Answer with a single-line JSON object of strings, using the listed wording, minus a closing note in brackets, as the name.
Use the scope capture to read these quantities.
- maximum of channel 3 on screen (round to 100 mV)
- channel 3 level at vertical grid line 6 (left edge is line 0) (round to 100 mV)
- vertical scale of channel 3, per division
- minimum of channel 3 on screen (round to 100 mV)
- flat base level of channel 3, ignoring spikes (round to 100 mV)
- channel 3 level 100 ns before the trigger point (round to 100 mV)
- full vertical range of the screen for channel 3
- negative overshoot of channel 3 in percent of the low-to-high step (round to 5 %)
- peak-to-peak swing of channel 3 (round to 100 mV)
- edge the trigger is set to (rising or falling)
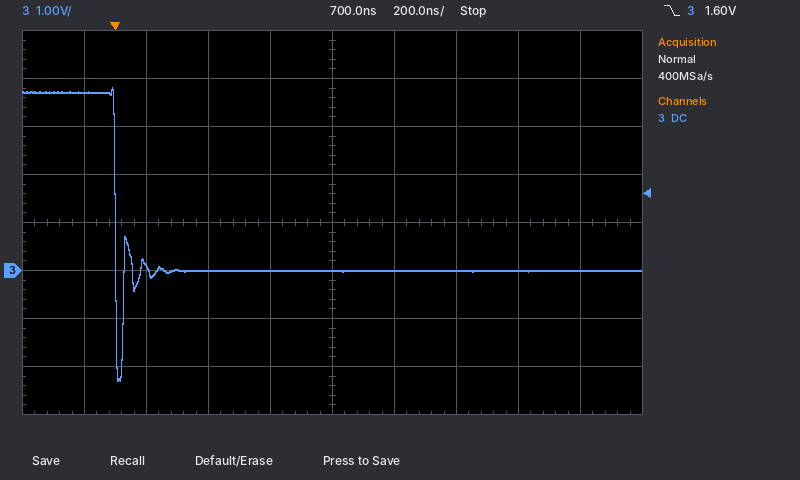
{"maximum of channel 3 on screen": "3.8 V", "channel 3 level at vertical grid line 6 (left edge is line 0)": "0.0 V", "vertical scale of channel 3, per division": "1 V", "minimum of channel 3 on screen": "-2.3 V", "flat base level of channel 3, ignoring spikes": "0.0 V", "channel 3 level 100 ns before the trigger point": "3.7 V", "full vertical range of the screen for channel 3": "8 V", "negative overshoot of channel 3 in percent of the low-to-high step": "60 %", "peak-to-peak swing of channel 3": "6.1 V", "edge the trigger is set to": "falling"}
